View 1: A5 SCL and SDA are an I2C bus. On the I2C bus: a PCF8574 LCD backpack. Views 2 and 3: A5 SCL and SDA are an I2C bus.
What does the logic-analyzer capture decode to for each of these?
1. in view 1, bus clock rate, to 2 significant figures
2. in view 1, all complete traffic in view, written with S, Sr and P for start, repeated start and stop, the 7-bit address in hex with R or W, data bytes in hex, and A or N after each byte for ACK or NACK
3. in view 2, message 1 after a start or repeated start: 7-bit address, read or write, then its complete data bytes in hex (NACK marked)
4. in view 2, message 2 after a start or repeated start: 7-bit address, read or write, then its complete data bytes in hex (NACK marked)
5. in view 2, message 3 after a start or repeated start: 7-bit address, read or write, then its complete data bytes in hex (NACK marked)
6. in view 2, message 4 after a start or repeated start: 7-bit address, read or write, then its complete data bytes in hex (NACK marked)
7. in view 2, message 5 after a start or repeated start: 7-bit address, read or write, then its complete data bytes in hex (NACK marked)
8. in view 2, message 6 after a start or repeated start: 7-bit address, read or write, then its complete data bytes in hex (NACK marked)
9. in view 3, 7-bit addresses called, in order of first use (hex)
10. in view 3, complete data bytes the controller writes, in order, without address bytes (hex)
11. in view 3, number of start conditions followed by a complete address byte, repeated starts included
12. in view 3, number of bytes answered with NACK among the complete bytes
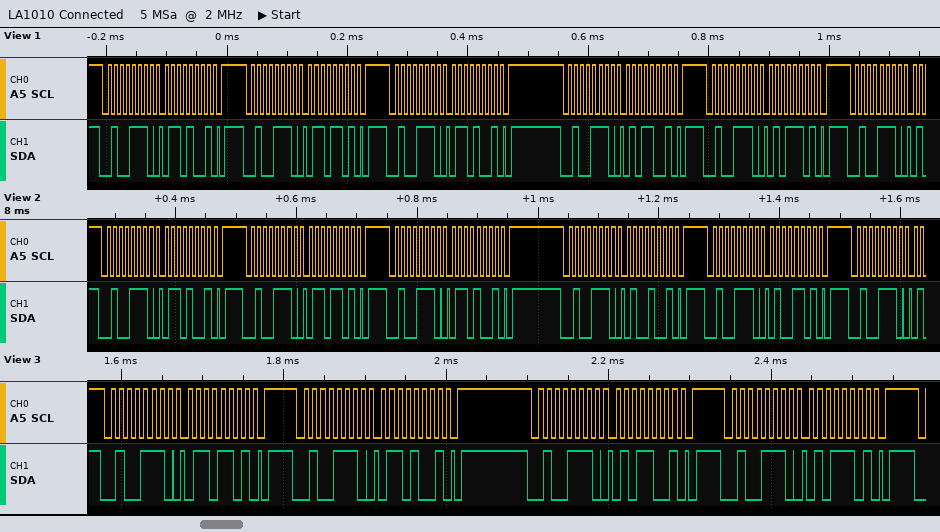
100 kHz
S 27W A 69 A P S 27W A 6D A P S 27W A 69 A P S 27W A 59 A P S 27W A 5D A P S 27W A
0x27 write: 69
0x27 write: 6D
0x27 write: 69
0x27 write: 49
0x27 write: 4D
0x27 write
0x27
6D 69 59 5D
4
0
